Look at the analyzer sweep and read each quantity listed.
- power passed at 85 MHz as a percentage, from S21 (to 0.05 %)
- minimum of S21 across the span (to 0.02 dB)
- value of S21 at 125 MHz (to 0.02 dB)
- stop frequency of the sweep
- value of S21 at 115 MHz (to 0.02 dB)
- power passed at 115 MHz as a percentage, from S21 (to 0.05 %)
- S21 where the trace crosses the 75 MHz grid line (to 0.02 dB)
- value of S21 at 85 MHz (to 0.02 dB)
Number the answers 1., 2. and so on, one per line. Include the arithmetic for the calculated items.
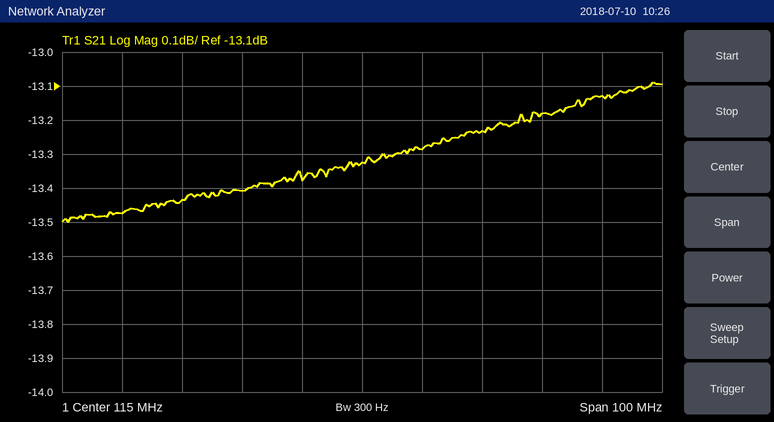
1. 10^(-13.44/10) ≈ 4.53 %, so 4.55 % to the nearest 0.05 %
2. -13.50 dB
3. -13.28 dB
4. 165 MHz
5. -13.32 dB
6. 10^(-13.32/10) ≈ 4.66 %, so 4.65 % to the nearest 0.05 %
7. -13.48 dB
8. -13.44 dB
